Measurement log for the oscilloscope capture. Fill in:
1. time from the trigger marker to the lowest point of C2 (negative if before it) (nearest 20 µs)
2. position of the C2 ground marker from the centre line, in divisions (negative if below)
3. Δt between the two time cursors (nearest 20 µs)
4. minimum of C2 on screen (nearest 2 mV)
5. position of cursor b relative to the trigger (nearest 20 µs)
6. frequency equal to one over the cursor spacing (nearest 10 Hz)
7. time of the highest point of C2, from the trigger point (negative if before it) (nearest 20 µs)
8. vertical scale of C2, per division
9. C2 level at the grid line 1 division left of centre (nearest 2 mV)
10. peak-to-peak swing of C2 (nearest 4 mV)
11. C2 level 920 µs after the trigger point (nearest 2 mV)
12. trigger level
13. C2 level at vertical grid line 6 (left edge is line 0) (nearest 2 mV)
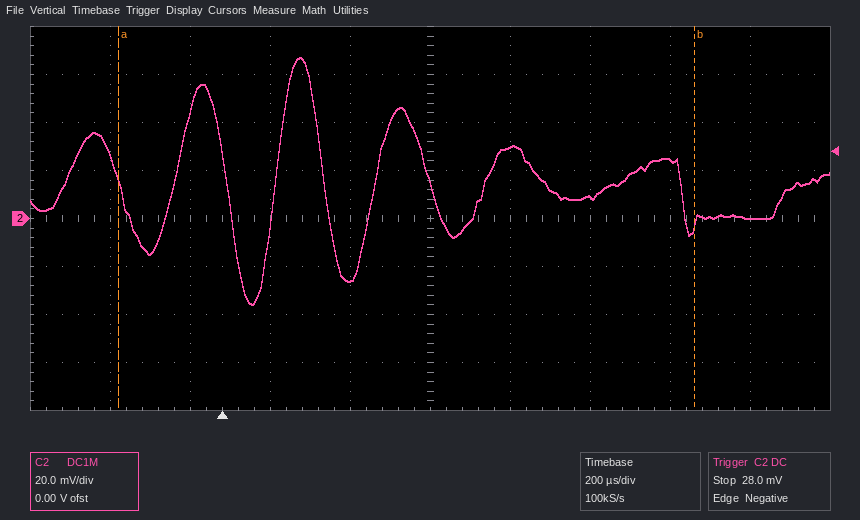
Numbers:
+80 µs
0.0 div
1.44 ms
-36 mV
+1.18 ms
690 Hz
+200 µs
20 mV
-26 mV
104 mV
8 mV
28.0 mV
30 mV
